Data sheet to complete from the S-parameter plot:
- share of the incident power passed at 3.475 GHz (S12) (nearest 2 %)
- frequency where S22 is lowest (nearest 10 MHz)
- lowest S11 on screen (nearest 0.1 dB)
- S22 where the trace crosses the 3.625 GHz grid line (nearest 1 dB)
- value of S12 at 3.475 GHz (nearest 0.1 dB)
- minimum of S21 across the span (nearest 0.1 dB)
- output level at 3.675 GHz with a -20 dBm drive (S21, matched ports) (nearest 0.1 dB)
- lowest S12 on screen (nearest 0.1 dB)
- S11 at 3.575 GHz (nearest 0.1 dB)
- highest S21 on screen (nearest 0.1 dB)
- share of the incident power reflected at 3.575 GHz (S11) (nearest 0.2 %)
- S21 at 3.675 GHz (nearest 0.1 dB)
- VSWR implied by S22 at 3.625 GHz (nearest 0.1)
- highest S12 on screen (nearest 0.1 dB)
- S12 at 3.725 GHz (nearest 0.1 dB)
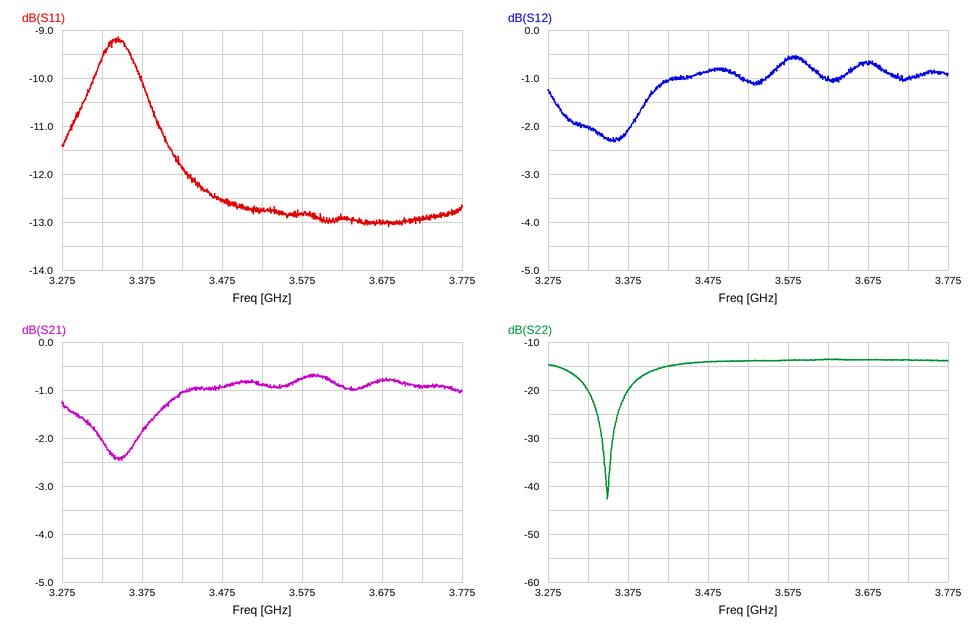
82 %
3.35 GHz
-13.1 dB
-14 dB
-0.9 dB
-2.5 dB
-20.8 dBm
-2.3 dB
-12.8 dB
-0.7 dB
5.2 %
-0.8 dB
1.5
-0.5 dB
-1.0 dB
